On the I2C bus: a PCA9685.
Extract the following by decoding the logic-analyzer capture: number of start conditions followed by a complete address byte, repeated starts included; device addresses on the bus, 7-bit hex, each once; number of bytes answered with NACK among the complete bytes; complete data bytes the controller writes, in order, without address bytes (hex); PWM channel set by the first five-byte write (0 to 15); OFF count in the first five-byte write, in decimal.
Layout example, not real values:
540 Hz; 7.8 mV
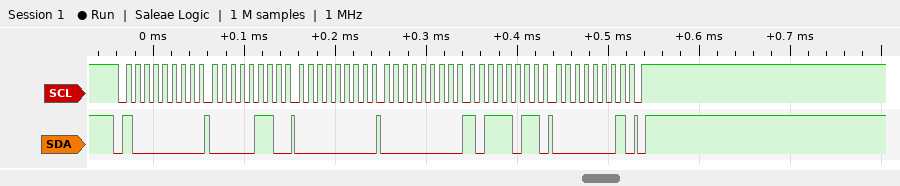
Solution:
1; 0x40; 0; 06 00 00 BB 01; 0; 443
